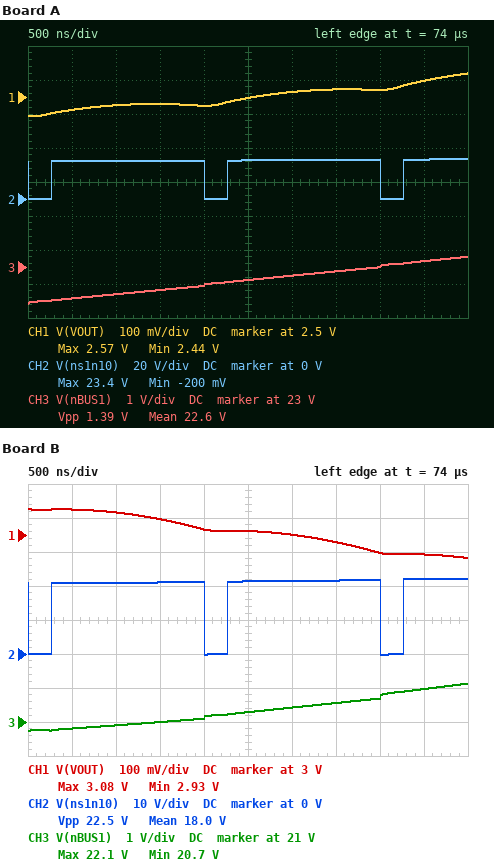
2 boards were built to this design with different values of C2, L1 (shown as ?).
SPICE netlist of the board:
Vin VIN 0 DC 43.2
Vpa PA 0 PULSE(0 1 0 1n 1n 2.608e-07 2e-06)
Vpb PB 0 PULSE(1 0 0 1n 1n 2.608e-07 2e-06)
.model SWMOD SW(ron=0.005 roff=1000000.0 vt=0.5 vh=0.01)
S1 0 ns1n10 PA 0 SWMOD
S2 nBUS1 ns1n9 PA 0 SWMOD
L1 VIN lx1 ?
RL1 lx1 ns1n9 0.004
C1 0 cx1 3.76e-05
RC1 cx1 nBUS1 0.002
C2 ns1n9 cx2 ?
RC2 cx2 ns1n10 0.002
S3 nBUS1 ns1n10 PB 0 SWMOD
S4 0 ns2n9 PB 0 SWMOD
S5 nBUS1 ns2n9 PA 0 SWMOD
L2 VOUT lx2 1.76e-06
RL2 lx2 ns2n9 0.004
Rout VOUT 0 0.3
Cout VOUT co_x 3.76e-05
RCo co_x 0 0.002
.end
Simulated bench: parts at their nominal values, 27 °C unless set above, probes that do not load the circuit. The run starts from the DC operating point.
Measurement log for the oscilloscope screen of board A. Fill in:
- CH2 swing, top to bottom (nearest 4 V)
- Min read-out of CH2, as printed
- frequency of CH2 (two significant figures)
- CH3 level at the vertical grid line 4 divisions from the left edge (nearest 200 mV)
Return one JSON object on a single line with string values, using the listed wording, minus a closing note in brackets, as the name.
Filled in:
{"CH2 swing, top to bottom": "24 V", "Min read-out of CH2, as printed": "-200 mV", "frequency of CH2": "500 kHz", "CH3 level at the vertical grid line 4 divisions from the left edge": "22.4 V"}
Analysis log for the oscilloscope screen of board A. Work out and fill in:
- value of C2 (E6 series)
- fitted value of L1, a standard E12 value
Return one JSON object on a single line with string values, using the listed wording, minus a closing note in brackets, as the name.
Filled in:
{"value of C2": "22 µF", "fitted value of L1, a standard E12 value": "5.6 µH"}
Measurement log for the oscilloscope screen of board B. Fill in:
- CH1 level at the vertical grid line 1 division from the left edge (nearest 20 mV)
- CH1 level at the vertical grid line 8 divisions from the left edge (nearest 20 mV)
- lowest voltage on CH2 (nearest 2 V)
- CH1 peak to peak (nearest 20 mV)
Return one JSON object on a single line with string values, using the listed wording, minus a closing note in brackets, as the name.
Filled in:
{"CH1 level at the vertical grid line 1 division from the left edge": "3.08 V", "CH1 level at the vertical grid line 8 divisions from the left edge": "2.94 V", "lowest voltage on CH2": "0 V", "CH1 peak to peak": "140 mV"}
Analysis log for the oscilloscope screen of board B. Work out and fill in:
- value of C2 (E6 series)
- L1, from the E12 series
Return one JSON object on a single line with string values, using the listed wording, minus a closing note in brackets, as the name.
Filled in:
{"value of C2": "15 µF", "L1, from the E12 series": "2.2 µH"}
